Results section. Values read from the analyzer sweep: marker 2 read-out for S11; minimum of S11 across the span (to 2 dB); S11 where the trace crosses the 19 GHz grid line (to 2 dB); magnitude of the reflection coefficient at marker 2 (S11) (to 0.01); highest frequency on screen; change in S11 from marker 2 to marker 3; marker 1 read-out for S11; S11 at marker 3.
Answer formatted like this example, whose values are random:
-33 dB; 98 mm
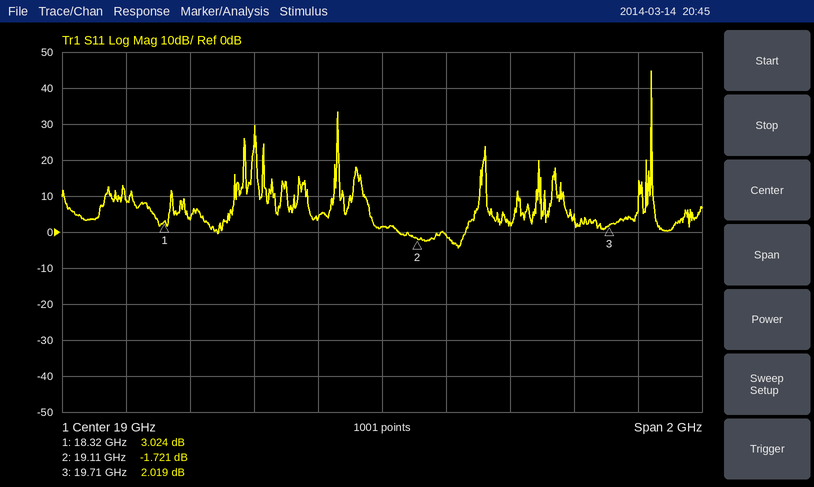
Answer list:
-1.721 dB; -4 dB; 2 dB; 0.82; 20 GHz; 3.740 dB; 3.024 dB; 2.019 dB
